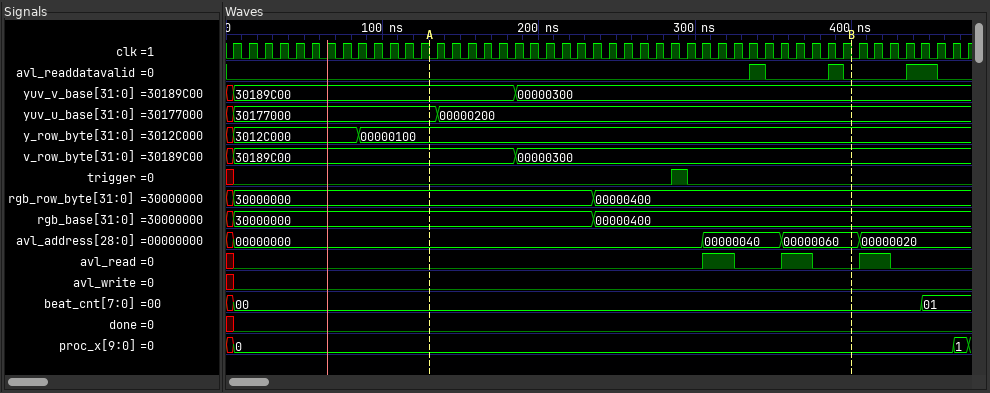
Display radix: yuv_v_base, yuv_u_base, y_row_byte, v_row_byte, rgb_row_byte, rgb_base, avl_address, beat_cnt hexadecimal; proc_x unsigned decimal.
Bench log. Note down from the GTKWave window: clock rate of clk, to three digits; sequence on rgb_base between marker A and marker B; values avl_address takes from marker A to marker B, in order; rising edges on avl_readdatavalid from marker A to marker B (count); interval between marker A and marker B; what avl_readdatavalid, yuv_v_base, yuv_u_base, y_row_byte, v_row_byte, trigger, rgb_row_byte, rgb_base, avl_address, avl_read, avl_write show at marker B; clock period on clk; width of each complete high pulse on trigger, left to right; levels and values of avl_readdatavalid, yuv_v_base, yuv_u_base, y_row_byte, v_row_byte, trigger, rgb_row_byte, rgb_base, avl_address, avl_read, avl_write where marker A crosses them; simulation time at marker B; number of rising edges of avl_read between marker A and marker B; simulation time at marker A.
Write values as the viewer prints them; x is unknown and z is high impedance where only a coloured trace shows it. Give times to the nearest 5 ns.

100 MHz
30000000, 00000400
00000000, 00000040, 00000060
2
270 ns
avl_readdatavalid=0, yuv_v_base=00000300, yuv_u_base=00000200, y_row_byte=00000100, v_row_byte=00000300, trigger=0, rgb_row_byte=00000400, rgb_base=00000400, avl_address=00000060, avl_read=0, avl_write=0
10 ns
10 ns
avl_readdatavalid=0, yuv_v_base=30189C00, yuv_u_base=30177000, y_row_byte=00000100, v_row_byte=30189C00, trigger=0, rgb_row_byte=30000000, rgb_base=30000000, avl_address=00000000, avl_read=0, avl_write=0
400 ns
2
130 ns
